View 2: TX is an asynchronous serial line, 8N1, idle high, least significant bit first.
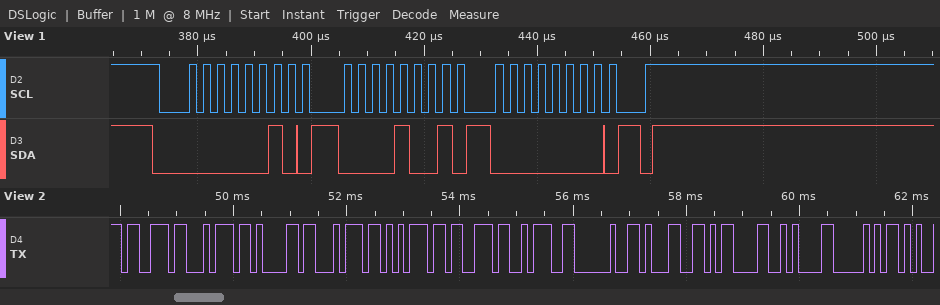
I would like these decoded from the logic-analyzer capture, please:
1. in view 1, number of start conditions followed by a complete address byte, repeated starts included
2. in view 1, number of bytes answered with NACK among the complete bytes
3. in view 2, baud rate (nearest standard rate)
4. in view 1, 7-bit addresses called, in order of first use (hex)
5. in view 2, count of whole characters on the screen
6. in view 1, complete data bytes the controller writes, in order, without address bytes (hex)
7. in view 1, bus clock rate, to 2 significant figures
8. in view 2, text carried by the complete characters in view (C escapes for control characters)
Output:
1
0
9600 baud
0x01
12
09 00
400 kHz
"status: 1\r\nP"
